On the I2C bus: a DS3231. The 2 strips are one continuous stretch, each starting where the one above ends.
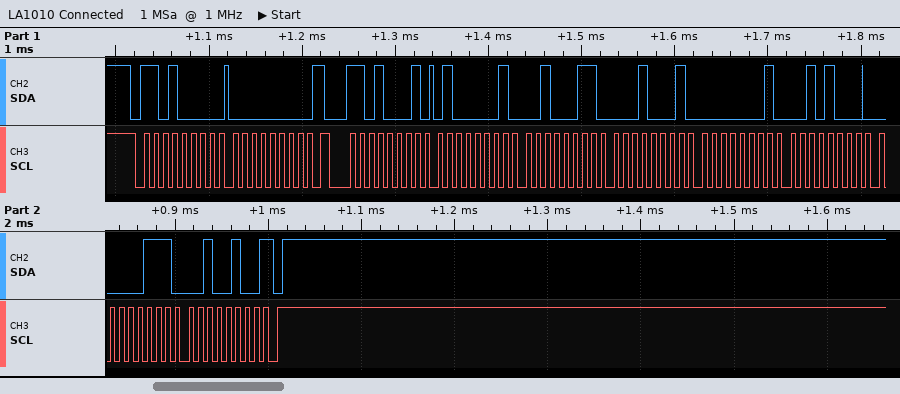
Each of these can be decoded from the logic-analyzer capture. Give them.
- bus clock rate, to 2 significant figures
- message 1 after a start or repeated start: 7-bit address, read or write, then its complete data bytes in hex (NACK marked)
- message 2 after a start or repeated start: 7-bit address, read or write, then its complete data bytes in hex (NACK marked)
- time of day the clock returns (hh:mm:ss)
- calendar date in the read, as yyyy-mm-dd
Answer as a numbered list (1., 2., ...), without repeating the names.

1. 100 kHz
2. 0x68 write: 00
3. 0x68 read: 41 23 11 01 28 07 24 NACK
4. 11:23:41
5. 2024-07-28
